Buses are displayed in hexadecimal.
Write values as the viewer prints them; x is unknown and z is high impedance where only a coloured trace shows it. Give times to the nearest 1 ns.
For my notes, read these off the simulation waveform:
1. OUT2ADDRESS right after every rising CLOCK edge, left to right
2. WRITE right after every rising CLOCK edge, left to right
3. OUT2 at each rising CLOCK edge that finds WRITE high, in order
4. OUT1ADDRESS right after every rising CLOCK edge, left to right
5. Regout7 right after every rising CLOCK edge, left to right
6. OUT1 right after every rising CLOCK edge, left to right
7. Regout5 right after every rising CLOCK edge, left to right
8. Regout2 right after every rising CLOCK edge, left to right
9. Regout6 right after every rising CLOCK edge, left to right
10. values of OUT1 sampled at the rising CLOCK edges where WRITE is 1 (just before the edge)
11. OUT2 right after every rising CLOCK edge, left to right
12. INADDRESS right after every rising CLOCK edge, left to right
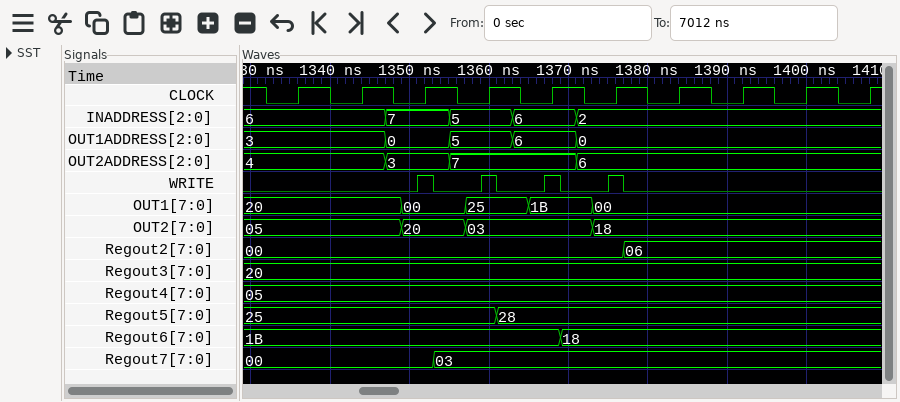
4, 4, 3, 7, 7, 6, 6, 6, 6, 6
0 0 1 1 1 1 0 0 0 0
20, 03, 03, 18
3, 3, 0, 5, 6, 0, 0, 0, 0, 0
00, 00, 00, 03, 03, 03, 03, 03, 03, 03
20, 20, 00, 25, 1B, 00, 00, 00, 00, 00
25, 25, 25, 25, 28, 28, 28, 28, 28, 28
00, 00, 00, 00, 00, 00, 06, 06, 06, 06
1B, 1B, 1B, 1B, 1B, 18, 18, 18, 18, 18
00, 25, 1B, 00
05, 05, 20, 03, 03, 18, 18, 18, 18, 18
6, 6, 7, 5, 6, 2, 2, 2, 2, 2
